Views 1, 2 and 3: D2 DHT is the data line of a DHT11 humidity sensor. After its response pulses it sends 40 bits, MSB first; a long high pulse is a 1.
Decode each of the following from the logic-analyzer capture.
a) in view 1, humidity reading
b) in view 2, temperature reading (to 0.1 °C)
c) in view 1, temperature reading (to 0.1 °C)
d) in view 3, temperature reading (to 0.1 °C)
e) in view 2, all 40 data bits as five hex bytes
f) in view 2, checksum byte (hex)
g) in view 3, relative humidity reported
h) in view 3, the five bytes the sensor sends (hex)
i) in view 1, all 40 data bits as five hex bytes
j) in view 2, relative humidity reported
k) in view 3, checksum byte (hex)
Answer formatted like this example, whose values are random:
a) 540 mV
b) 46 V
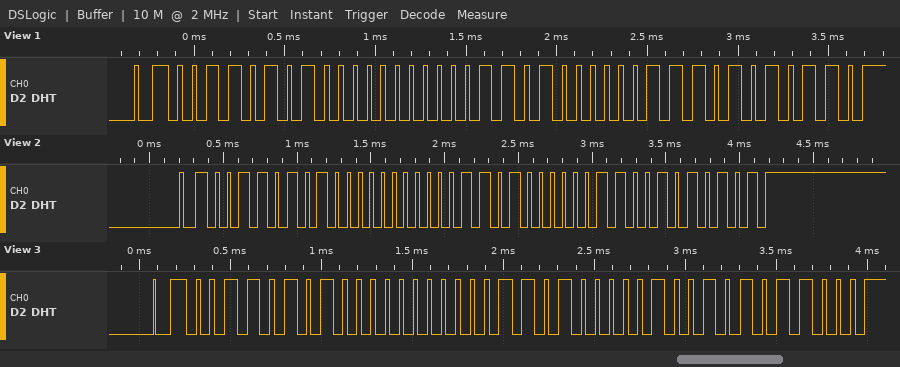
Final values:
a) 53 %
b) 26.6 °C
c) 26.7 °C
d) 26.9 °C
e) 35 00 1A 06 55
f) 0x55
g) 53 %
h) 35 00 1A 09 58
i) 35 00 1A 07 56
j) 53 %
k) 0x58
